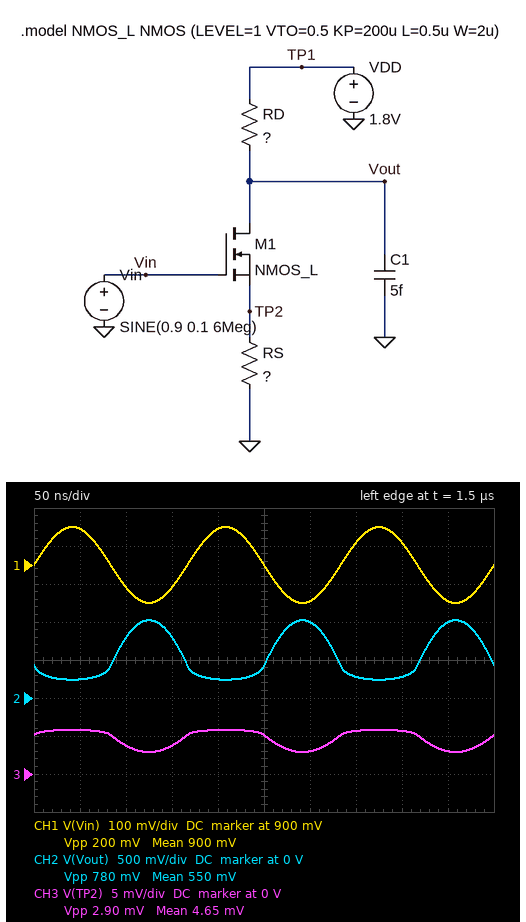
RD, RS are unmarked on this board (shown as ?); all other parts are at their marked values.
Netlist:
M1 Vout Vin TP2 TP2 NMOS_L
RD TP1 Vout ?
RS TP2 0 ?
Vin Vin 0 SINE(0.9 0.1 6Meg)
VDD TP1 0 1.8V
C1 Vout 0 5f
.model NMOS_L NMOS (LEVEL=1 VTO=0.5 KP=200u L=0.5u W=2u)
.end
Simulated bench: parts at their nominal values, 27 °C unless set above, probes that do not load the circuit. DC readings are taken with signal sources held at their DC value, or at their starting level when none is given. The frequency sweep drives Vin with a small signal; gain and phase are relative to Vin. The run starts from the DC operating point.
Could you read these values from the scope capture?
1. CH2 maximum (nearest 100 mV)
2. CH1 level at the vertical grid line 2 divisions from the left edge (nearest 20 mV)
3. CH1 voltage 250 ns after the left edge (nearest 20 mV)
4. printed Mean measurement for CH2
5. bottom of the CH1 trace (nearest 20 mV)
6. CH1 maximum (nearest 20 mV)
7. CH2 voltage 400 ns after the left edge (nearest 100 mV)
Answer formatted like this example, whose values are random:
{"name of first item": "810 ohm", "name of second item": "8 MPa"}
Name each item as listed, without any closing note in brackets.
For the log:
{"CH2 maximum": "1.0 V", "CH1 level at the vertical grid line 2 divisions from the left edge": "840 mV", "CH1 voltage 250 ns after the left edge": "900 mV", "printed Mean measurement for CH2": "550 mV", "bottom of the CH1 trace": "800 mV", "CH1 maximum": "1.00 V", "CH2 voltage 400 ns after the left edge": "300 mV"}
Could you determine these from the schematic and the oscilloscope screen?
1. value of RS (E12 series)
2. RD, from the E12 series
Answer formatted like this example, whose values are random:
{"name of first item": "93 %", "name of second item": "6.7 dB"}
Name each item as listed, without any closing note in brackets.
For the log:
{"value of RS": "82 Ω", "RD, from the E12 series": "22 kΩ"}
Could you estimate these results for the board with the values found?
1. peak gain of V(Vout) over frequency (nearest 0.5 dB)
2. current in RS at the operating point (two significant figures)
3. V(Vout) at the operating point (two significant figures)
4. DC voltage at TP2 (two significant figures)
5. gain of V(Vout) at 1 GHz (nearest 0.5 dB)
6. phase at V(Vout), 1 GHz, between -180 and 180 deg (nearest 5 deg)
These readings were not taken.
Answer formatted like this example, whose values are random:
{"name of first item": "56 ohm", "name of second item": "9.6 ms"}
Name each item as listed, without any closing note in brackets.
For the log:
{"peak gain of V(Vout) over frequency": "16.5 dB", "current in RS at the operating point": "62 µA", "V(Vout) at the operating point": "430 mV", "DC voltage at TP2": "5.1 mV", "gain of V(Vout) at 1 GHz": "15.0 dB", "phase at V(Vout), 1 GHz, between -180 and 180 deg": "145 deg"}
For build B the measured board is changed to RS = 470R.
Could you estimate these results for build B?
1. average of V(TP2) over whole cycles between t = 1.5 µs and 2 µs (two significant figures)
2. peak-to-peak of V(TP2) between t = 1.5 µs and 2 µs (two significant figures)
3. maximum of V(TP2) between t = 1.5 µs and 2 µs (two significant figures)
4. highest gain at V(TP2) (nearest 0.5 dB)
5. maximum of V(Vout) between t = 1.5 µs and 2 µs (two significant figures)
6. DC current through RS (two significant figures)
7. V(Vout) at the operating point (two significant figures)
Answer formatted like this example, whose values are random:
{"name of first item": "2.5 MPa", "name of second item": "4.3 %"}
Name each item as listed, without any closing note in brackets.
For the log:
{"average of V(TP2) over whole cycles between t = 1.5 µs and 2 µs": "25 mV", "peak-to-peak of V(TP2) between t = 1.5 µs and 2 µs": "17 mV", "maximum of V(TP2) between t = 1.5 µs and 2 µs": "32 mV", "highest gain at V(TP2)": "-18.0 dB", "maximum of V(Vout) between t = 1.5 µs and 2 µs": "1.1 V", "DC current through RS": "56 µA", "V(Vout) at the operating point": "570 mV"}
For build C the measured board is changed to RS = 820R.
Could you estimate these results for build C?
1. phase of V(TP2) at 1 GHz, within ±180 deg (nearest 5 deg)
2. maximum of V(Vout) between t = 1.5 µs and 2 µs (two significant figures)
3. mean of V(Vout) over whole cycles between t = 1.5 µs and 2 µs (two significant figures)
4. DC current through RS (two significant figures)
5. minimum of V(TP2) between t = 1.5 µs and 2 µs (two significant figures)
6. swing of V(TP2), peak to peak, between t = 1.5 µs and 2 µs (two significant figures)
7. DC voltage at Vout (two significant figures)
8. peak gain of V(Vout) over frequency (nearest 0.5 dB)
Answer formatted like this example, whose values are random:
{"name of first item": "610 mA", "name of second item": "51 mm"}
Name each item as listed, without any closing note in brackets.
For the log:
{"phase of V(TP2) at 1 GHz, within ±180 deg": "0 deg", "maximum of V(Vout) between t = 1.5 µs and 2 µs": "1.1 V", "mean of V(Vout) over whole cycles between t = 1.5 µs and 2 µs": "690 mV", "DC current through RS": "51 µA", "minimum of V(TP2) between t = 1.5 µs and 2 µs": "25 mV", "swing of V(TP2), peak to peak, between t = 1.5 µs and 2 µs": "30 mV", "DC voltage at Vout": "670 mV", "peak gain of V(Vout) over frequency": "14.0 dB"}
